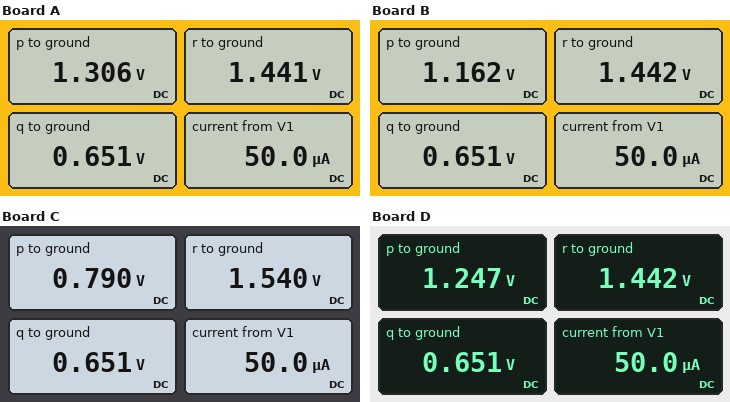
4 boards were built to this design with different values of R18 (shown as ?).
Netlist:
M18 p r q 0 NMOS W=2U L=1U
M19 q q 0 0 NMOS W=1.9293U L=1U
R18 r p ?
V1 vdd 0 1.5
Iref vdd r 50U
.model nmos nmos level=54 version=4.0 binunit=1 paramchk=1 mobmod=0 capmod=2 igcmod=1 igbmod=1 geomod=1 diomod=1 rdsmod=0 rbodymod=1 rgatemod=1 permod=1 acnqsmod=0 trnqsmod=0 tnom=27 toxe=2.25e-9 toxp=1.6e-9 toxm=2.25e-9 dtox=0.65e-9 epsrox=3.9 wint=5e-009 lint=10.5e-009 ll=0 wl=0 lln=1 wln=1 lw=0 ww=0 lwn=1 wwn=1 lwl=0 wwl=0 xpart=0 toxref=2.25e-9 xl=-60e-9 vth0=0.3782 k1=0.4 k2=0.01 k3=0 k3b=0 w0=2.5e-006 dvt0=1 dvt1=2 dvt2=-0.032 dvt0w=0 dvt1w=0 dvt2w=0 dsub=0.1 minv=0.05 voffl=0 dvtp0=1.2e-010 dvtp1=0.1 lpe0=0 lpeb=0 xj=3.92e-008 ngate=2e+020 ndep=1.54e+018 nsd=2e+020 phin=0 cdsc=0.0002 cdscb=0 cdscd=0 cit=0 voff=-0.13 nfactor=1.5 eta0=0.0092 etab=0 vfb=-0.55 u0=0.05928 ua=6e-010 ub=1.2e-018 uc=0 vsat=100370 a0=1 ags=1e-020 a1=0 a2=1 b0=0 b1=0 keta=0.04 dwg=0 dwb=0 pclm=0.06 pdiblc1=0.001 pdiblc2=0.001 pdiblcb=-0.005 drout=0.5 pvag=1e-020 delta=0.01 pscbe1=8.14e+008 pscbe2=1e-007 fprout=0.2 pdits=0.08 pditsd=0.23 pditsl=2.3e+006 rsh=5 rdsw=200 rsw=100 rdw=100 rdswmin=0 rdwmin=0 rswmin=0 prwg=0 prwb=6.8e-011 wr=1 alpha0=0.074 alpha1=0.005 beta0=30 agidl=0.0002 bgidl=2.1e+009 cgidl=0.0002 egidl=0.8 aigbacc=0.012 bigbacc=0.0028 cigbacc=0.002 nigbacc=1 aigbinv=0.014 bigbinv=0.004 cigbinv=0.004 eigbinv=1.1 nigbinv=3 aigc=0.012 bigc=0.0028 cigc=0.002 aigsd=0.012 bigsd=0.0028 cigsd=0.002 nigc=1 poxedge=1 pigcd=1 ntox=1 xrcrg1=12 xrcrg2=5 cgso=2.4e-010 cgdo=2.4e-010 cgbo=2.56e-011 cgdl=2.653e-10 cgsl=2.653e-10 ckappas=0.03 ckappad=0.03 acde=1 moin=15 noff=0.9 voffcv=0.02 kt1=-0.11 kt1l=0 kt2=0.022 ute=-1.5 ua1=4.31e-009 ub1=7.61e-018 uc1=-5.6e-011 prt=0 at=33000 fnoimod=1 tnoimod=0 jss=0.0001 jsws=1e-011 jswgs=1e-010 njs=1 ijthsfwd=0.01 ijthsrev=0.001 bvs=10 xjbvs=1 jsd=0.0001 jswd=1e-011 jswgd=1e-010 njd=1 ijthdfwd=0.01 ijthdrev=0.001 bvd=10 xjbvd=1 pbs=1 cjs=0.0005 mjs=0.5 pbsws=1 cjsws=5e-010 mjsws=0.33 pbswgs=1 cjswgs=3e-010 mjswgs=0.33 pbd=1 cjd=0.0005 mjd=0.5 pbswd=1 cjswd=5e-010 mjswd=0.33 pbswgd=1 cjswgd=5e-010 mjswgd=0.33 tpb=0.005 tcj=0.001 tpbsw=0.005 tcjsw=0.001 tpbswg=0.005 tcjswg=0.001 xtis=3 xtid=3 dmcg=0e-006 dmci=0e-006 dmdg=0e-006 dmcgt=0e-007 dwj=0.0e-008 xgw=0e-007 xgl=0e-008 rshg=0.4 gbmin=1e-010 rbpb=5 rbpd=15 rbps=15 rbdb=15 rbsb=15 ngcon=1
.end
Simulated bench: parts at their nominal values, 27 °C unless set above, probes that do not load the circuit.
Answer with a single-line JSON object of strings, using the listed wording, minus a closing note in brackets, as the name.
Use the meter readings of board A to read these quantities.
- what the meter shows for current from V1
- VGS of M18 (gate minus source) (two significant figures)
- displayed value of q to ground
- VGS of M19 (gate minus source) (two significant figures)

{"what the meter shows for current from V1": "50.0 µA", "VGS of M18 (gate minus source)": "790 mV", "displayed value of q to ground": "0.651 V", "VGS of M19 (gate minus source)": "650 mV"}
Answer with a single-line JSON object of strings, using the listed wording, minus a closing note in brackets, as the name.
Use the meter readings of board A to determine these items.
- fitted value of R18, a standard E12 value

{"fitted value of R18, a standard E12 value": "2.7 kΩ"}
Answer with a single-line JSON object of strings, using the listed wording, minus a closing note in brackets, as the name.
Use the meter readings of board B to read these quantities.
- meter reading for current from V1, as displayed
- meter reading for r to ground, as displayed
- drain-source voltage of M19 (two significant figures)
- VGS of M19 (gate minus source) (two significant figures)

{"meter reading for current from V1, as displayed": "50.0 µA", "meter reading for r to ground, as displayed": "1.442 V", "drain-source voltage of M19": "650 mV", "VGS of M19 (gate minus source)": "650 mV"}
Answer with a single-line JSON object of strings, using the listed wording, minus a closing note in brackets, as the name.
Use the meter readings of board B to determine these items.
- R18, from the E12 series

{"R18, from the E12 series": "5.6 kΩ"}
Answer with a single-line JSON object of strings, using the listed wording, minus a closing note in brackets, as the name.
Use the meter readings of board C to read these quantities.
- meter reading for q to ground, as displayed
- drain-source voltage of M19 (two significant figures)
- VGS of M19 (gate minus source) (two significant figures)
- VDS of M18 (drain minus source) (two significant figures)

{"meter reading for q to ground, as displayed": "0.651 V", "drain-source voltage of M19": "650 mV", "VGS of M19 (gate minus source)": "650 mV", "VDS of M18 (drain minus source)": "140 mV"}
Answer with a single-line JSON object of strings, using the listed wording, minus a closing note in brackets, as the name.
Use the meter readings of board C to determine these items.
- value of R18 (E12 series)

{"value of R18": "15 kΩ"}
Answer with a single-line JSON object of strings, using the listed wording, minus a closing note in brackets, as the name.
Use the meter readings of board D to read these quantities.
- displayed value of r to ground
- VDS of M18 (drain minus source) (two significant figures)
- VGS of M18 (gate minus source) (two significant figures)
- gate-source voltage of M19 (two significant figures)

{"displayed value of r to ground": "1.442 V", "VDS of M18 (drain minus source)": "600 mV", "VGS of M18 (gate minus source)": "790 mV", "gate-source voltage of M19": "650 mV"}
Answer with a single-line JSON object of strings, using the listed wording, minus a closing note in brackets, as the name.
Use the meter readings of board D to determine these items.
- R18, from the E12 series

{"R18, from the E12 series": "3.9 kΩ"}
